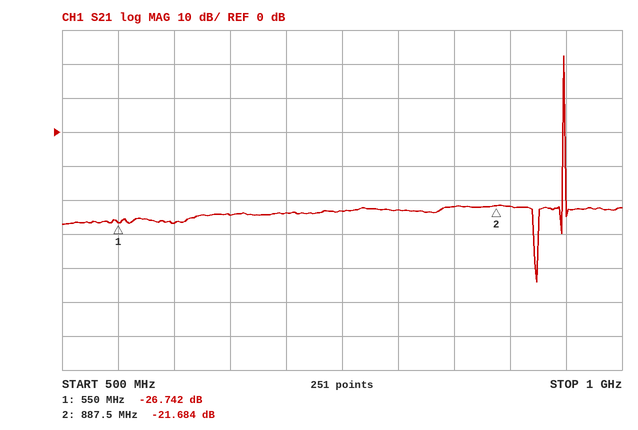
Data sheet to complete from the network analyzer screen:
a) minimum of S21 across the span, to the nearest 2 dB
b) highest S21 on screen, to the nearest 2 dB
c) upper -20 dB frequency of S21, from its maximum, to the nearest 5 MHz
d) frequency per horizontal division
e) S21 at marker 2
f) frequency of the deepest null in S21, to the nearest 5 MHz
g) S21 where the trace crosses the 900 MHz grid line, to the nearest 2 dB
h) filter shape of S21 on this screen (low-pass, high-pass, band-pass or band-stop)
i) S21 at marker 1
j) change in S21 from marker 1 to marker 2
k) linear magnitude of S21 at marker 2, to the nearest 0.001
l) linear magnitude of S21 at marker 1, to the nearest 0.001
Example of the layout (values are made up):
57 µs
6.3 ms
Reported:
-44 dB
22 dB
950 MHz
50 MHz
-21.684 dB
925 MHz
-22 dB
band-pass
-26.742 dB
5.058 dB
0.082
0.046
